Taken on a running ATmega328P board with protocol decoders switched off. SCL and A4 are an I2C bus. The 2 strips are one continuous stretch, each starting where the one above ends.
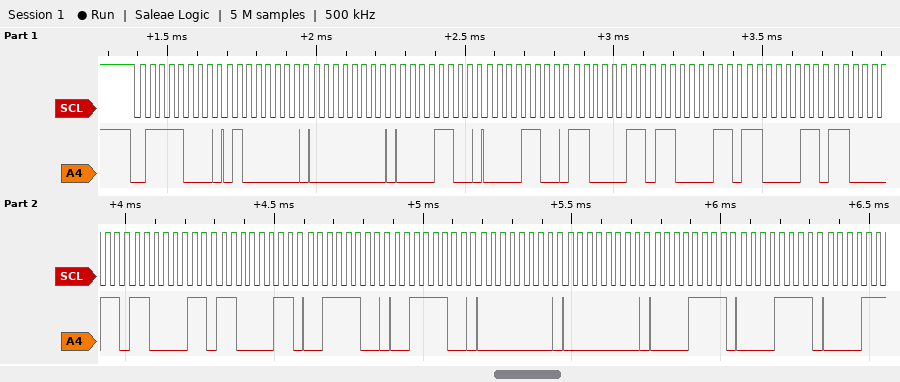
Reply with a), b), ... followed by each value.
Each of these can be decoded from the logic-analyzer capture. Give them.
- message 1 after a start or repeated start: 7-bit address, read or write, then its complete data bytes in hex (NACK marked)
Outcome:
a) 0x3C write: 40 00 0C 0C C3 C3 C3 C3 C3 C3 3C 3C 00 00 0F 0F
